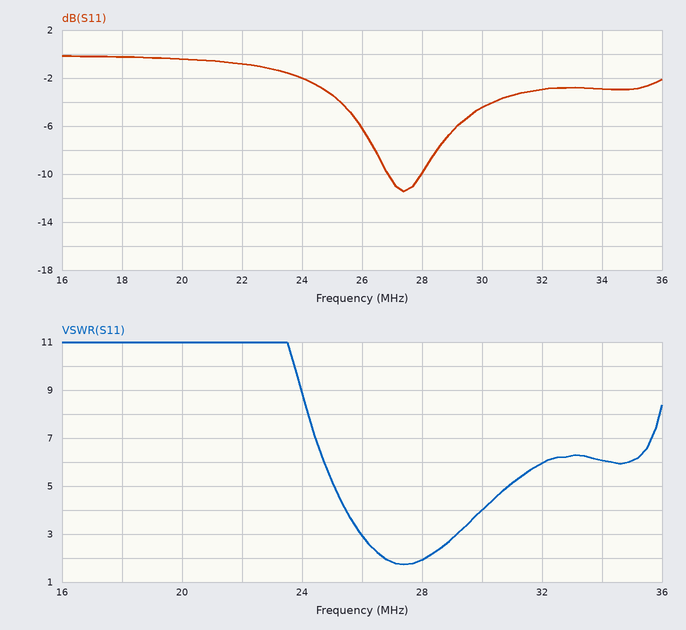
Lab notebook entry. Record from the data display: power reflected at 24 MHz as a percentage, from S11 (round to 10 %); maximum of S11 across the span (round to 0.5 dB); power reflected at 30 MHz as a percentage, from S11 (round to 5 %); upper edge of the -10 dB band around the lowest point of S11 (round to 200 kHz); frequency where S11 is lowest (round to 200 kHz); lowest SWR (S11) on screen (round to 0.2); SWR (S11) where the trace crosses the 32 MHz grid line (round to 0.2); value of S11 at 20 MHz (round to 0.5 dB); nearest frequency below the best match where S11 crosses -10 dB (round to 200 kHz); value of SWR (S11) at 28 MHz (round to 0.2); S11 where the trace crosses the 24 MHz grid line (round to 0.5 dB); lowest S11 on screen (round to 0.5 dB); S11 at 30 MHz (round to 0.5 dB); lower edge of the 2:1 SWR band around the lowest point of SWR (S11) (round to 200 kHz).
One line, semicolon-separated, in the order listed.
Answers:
60 %; 0.0 dB; 35 %; 28.0 MHz; 27.4 MHz; 1.8; 6.0; -0.5 dB; 26.8 MHz; 2.0; -2.0 dB; -11.5 dB; -4.5 dB; 26.8 MHz
